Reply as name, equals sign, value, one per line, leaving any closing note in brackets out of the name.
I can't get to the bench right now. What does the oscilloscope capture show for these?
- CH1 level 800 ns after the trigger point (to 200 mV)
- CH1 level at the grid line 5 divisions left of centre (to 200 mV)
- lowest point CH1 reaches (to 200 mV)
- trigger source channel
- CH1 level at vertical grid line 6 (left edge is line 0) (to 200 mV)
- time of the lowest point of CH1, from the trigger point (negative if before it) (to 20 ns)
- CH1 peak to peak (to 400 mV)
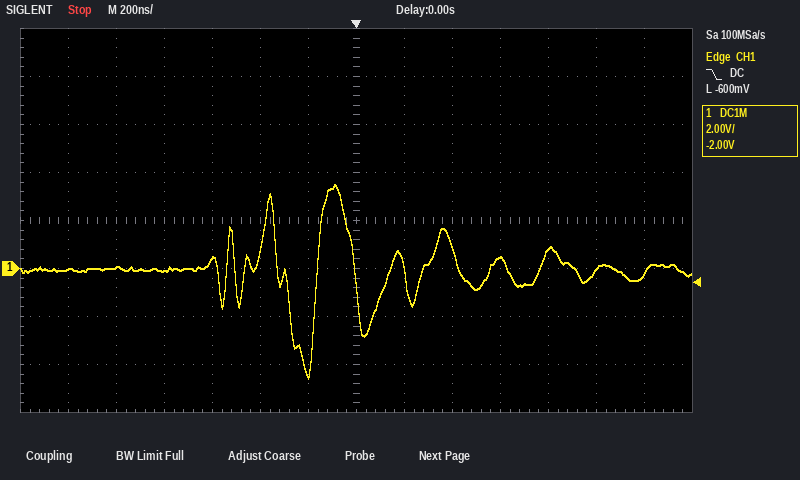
CH1 level 800 ns after the trigger point = 800 mV
CH1 level at the grid line 5 divisions left of centre = 0.0 V
lowest point CH1 reaches = -4.6 V
trigger source channel = CH1
CH1 level at vertical grid line 6 (left edge is line 0) = -4.4 V
time of the lowest point of CH1, from the trigger point (negative if before it) = -200 ns
CH1 peak to peak = 8.0 V
